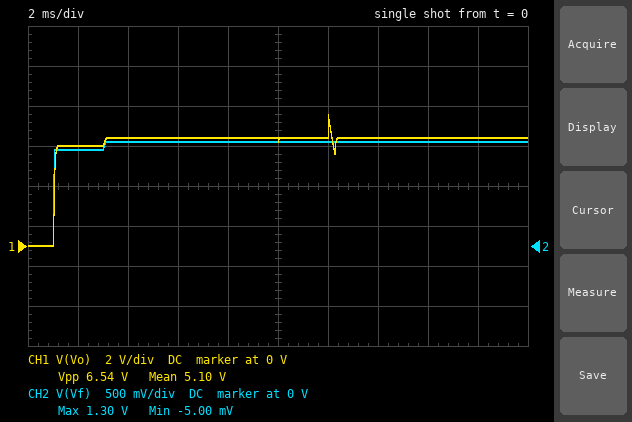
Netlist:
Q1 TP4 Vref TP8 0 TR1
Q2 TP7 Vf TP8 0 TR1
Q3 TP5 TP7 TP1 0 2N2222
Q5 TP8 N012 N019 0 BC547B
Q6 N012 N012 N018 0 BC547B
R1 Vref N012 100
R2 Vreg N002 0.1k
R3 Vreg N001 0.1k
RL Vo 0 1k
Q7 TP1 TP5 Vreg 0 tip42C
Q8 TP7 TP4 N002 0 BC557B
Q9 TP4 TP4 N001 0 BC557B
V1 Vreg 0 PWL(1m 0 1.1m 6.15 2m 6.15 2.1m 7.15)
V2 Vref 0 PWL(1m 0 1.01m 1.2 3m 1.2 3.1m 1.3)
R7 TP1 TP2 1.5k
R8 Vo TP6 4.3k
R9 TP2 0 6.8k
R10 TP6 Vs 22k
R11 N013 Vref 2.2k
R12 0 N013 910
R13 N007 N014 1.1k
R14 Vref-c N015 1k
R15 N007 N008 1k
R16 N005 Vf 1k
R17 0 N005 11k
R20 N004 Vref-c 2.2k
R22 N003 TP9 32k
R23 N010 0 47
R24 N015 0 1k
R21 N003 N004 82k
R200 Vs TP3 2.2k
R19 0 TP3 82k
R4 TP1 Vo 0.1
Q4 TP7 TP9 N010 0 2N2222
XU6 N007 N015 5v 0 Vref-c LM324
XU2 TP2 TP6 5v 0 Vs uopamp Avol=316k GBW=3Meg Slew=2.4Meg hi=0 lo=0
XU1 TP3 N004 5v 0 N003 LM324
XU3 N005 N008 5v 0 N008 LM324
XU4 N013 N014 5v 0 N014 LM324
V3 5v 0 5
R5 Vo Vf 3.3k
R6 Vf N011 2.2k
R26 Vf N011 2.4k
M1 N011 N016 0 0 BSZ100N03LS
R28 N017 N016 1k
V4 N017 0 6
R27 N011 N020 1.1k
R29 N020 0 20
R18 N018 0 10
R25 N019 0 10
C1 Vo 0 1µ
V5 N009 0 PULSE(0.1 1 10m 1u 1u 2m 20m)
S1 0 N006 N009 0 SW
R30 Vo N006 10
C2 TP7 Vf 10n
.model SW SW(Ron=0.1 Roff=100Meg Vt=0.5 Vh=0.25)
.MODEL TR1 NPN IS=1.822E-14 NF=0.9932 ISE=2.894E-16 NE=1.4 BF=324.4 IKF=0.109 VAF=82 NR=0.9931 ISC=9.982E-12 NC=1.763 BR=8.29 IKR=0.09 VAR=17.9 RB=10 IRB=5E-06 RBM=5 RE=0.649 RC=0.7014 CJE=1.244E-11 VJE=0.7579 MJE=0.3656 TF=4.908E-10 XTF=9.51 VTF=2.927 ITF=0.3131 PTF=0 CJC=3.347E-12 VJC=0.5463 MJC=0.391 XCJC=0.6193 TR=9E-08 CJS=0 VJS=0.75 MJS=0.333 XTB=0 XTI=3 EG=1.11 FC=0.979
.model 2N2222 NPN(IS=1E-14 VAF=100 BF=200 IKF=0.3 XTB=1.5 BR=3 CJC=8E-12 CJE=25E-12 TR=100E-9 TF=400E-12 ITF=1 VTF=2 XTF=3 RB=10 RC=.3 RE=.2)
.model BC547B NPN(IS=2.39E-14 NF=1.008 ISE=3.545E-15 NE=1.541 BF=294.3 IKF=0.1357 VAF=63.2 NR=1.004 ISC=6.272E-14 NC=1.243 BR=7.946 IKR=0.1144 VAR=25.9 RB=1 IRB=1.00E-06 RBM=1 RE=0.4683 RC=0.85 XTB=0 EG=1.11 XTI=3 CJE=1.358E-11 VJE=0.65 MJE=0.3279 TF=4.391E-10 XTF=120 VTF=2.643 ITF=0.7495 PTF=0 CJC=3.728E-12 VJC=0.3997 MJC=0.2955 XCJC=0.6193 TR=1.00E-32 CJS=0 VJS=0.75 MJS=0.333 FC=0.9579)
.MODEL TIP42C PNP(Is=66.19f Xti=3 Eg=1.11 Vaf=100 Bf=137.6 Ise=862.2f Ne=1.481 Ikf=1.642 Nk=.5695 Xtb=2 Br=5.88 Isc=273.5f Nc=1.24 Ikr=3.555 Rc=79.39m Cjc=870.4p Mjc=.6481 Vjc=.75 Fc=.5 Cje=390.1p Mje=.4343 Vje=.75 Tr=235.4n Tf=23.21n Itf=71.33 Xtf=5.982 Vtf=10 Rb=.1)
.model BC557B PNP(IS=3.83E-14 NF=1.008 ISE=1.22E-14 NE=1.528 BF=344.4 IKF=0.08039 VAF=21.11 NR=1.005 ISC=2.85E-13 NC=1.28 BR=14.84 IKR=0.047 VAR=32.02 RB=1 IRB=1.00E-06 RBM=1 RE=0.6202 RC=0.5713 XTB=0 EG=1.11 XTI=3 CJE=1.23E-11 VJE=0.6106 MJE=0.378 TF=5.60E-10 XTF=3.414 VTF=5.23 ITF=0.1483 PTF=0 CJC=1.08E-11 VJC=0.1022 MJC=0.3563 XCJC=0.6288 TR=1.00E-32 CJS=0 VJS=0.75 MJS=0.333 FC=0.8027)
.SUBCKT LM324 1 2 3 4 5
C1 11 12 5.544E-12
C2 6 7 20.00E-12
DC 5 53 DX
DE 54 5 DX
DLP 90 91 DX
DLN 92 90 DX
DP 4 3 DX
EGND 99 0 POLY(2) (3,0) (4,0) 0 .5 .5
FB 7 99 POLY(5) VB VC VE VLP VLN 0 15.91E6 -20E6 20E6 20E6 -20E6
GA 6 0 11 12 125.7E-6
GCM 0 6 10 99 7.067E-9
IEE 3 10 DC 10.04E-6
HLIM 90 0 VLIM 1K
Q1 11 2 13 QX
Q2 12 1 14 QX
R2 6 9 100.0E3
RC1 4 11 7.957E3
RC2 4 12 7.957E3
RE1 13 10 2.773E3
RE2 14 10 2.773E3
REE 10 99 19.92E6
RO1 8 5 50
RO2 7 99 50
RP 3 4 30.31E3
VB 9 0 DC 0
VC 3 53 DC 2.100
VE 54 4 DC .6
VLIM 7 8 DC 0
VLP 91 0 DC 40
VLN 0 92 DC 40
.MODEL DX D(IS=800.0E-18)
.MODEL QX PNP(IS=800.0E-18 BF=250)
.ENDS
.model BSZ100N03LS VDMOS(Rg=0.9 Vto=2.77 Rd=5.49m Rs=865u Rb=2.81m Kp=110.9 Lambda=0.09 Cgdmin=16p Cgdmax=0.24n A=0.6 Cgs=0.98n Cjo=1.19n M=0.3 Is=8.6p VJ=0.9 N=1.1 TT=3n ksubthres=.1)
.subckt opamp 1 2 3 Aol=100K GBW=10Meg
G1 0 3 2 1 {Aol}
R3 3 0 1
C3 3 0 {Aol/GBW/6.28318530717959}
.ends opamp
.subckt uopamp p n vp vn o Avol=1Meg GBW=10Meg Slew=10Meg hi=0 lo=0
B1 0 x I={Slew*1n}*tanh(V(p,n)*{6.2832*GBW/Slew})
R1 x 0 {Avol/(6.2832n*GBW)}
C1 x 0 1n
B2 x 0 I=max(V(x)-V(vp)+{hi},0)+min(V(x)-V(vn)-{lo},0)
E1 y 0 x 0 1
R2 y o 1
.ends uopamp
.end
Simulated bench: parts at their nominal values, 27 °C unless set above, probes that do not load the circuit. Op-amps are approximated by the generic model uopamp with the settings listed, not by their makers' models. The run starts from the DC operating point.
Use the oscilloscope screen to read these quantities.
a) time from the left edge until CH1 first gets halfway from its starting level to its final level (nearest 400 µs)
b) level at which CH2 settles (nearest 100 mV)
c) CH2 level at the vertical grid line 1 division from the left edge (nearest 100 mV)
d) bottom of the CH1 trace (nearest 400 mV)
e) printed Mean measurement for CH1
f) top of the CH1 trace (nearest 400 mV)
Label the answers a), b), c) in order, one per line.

a) 1.2 ms
b) 1.3 V
c) 1.2 V
d) 0 V
e) 5.10 V
f) 6.4 V
